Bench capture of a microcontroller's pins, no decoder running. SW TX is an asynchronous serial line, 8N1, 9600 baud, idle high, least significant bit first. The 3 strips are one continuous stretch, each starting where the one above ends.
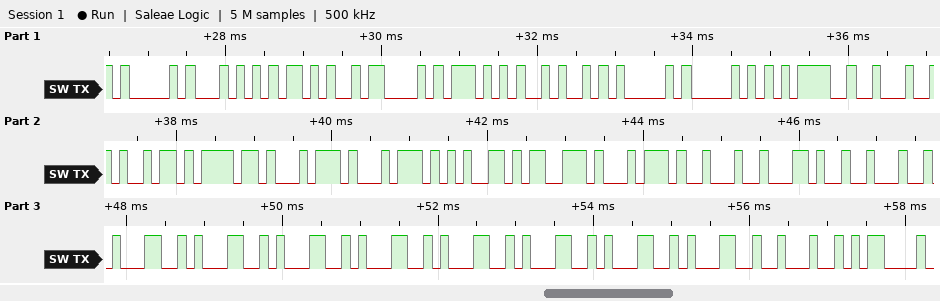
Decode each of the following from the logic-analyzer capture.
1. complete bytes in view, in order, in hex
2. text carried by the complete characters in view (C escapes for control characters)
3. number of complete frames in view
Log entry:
41 54 2B 43 57 4A 41 50 3D 22 69 6F 74 74 65 73 74 22 2C 22 31 31 31 31 31 31 31 31 22 0D
"AT+CWJAP=\"iottest\",\"11111111\"\r"
30
